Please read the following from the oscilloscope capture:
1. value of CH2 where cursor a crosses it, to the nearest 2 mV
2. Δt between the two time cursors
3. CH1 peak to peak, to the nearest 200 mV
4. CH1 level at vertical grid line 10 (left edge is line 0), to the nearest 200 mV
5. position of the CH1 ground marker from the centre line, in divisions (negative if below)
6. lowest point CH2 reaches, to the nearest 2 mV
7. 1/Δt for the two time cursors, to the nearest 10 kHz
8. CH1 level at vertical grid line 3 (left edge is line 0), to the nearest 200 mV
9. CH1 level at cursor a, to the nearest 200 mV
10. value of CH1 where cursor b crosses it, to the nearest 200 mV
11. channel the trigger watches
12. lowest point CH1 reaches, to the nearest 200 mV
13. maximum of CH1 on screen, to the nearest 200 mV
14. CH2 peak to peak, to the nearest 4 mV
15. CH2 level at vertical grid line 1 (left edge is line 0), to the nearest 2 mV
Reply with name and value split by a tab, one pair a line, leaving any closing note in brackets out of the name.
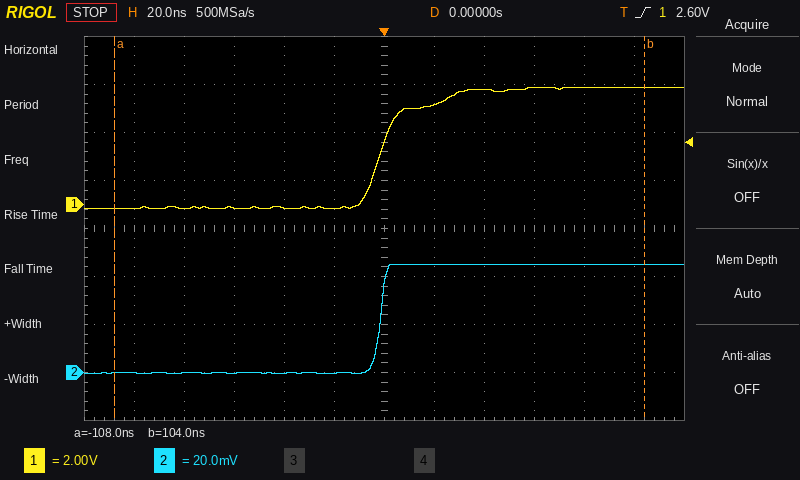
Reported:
value of CH2 where cursor a crosses it, to the nearest 2 mV	0 mV
Δt between the two time cursors	212 ns
CH1 peak to peak, to the nearest 200 mV	5.0 V
CH1 level at vertical grid line 10 (left edge is line 0), to the nearest 200 mV	4.8 V
position of the CH1 ground marker from the centre line, in divisions	+0.5 div
lowest point CH2 reaches, to the nearest 2 mV	0 mV
1/Δt for the two time cursors, to the nearest 10 kHz	4.72 MHz
CH1 level at vertical grid line 3 (left edge is line 0), to the nearest 200 mV	-200 mV
CH1 level at cursor a, to the nearest 200 mV	-200 mV
value of CH1 where cursor b crosses it, to the nearest 200 mV	4.8 V
channel the trigger watches	CH1
lowest point CH1 reaches, to the nearest 200 mV	-200 mV
maximum of CH1 on screen, to the nearest 200 mV	4.8 V
CH2 peak to peak, to the nearest 4 mV	44 mV
CH2 level at vertical grid line 1 (left edge is line 0), to the nearest 2 mV	0 mV
